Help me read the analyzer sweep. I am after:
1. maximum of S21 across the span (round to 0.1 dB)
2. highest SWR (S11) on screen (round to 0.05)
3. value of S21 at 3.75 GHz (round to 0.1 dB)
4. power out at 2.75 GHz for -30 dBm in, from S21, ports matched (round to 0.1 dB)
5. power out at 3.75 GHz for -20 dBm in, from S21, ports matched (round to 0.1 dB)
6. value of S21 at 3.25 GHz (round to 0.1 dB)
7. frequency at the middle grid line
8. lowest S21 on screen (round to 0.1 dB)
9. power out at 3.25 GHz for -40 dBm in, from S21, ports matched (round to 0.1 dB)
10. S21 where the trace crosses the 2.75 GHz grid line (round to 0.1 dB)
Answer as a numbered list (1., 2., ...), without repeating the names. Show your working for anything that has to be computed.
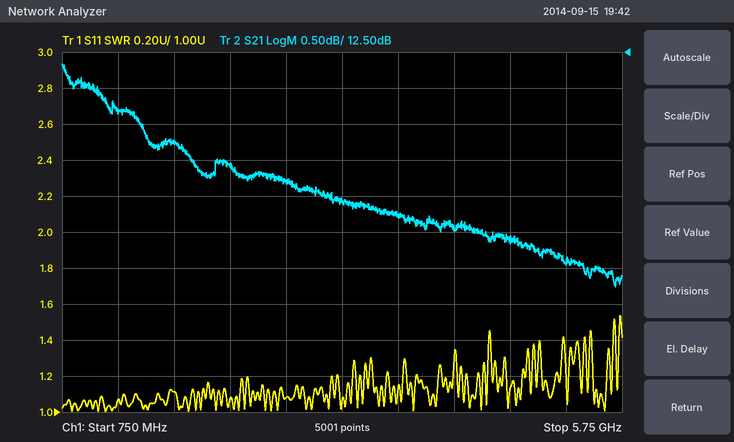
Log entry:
1. 12.3 dB
2. 1.55
3. 10.2 dB
4. -30 dBm + (10.7 dB) = -19.3 dBm
5. -20 dBm + (10.2 dB) = -9.8 dBm
6. 10.4 dB
7. 3.25 GHz
8. 9.2 dB
9. -40 dBm + (10.4 dB) = -29.6 dBm
10. 10.7 dB
